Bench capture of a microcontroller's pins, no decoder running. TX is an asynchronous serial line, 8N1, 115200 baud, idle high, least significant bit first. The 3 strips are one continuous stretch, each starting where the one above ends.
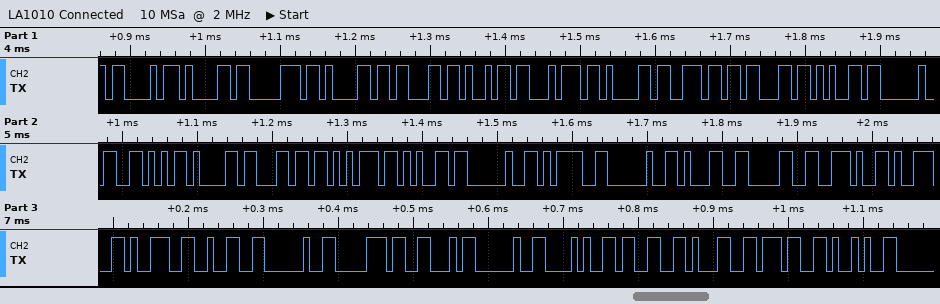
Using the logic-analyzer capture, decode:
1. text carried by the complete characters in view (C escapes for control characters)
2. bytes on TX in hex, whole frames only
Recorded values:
"Capacitance Value = 10.992 pF (317)"
43 61 70 61 63 69 74 61 6E 63 65 20 56 61 6C 75 65 20 3D 20 31 30 2E 39 39 32 20 70 46 20 28 33 31 37 29
